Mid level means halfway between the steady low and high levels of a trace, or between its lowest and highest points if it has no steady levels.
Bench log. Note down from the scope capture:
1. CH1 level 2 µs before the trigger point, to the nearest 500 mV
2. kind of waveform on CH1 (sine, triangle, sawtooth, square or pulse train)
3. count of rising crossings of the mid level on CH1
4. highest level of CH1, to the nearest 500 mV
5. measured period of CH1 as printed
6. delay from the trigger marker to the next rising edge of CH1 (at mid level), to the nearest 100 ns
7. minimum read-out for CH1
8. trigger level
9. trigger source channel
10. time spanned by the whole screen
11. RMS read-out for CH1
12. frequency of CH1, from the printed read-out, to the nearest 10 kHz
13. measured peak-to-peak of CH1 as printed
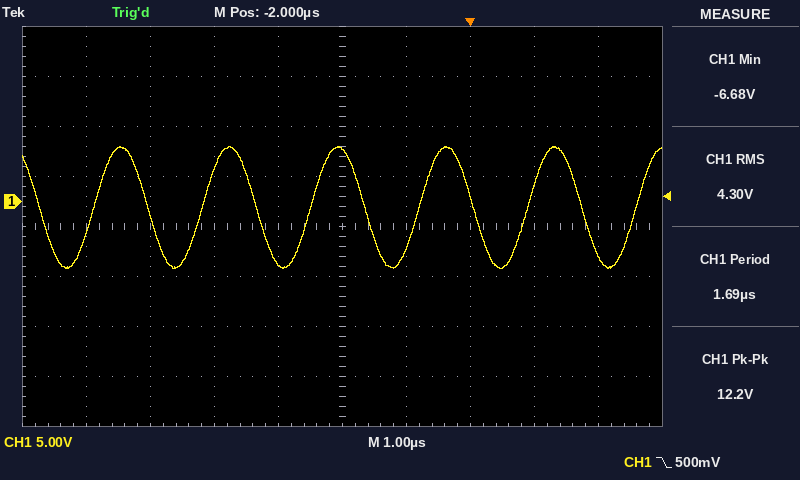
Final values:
5.0 V
sine
6
5.5 V
1.69 µs
900 ns
-6.68 V
500 mV
CH1
10 µs
4.30 V
590 kHz
12.2 V
